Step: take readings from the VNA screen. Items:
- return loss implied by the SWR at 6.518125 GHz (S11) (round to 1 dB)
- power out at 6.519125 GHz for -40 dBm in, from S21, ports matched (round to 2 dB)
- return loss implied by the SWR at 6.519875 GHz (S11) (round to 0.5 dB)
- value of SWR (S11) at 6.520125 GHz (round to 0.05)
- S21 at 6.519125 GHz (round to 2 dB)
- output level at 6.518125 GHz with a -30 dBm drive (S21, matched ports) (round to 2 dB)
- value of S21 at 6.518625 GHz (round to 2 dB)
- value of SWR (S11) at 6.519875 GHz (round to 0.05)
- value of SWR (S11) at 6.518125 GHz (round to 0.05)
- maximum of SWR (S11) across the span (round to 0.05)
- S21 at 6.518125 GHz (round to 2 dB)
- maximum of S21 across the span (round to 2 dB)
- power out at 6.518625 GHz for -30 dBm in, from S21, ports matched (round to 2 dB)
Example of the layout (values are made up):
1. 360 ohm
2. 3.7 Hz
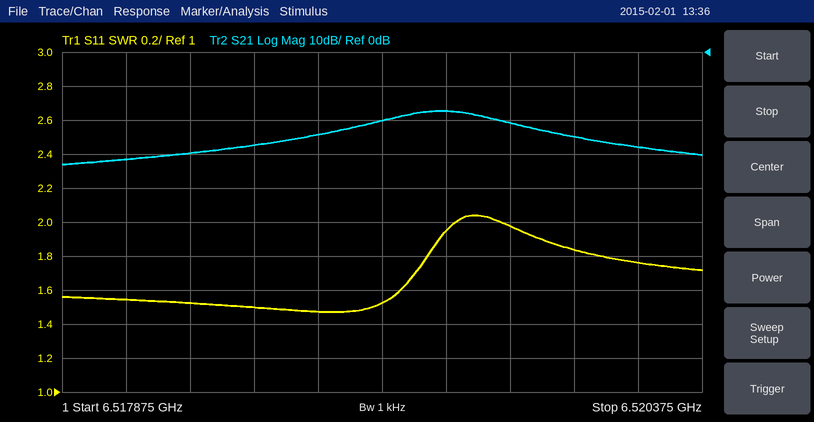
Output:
1. 13 dB
2. -60 dBm
3. 10.5 dB
4. 1.75
5. -20 dB
6. -62 dBm
7. -28 dB
8. 1.85
9. 1.55
10. 2.05
11. -32 dB
12. -18 dB
13. -58 dBm
